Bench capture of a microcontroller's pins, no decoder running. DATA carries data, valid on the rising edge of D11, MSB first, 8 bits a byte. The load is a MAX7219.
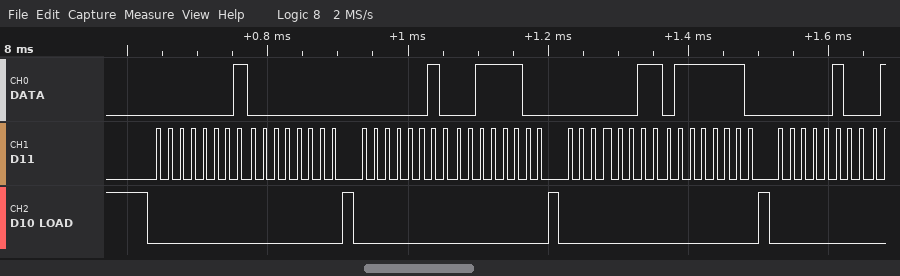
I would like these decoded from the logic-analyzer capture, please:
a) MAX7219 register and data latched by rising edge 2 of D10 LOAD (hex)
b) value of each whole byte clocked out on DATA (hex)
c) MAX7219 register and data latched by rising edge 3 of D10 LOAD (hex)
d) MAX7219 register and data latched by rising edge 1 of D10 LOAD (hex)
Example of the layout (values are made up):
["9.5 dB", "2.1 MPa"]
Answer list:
["register 0x2, data 0x3C", "01 00 02 3C 03 7E 04", "register 0x3, data 0x7E", "register 0x1, data 0x00"]
